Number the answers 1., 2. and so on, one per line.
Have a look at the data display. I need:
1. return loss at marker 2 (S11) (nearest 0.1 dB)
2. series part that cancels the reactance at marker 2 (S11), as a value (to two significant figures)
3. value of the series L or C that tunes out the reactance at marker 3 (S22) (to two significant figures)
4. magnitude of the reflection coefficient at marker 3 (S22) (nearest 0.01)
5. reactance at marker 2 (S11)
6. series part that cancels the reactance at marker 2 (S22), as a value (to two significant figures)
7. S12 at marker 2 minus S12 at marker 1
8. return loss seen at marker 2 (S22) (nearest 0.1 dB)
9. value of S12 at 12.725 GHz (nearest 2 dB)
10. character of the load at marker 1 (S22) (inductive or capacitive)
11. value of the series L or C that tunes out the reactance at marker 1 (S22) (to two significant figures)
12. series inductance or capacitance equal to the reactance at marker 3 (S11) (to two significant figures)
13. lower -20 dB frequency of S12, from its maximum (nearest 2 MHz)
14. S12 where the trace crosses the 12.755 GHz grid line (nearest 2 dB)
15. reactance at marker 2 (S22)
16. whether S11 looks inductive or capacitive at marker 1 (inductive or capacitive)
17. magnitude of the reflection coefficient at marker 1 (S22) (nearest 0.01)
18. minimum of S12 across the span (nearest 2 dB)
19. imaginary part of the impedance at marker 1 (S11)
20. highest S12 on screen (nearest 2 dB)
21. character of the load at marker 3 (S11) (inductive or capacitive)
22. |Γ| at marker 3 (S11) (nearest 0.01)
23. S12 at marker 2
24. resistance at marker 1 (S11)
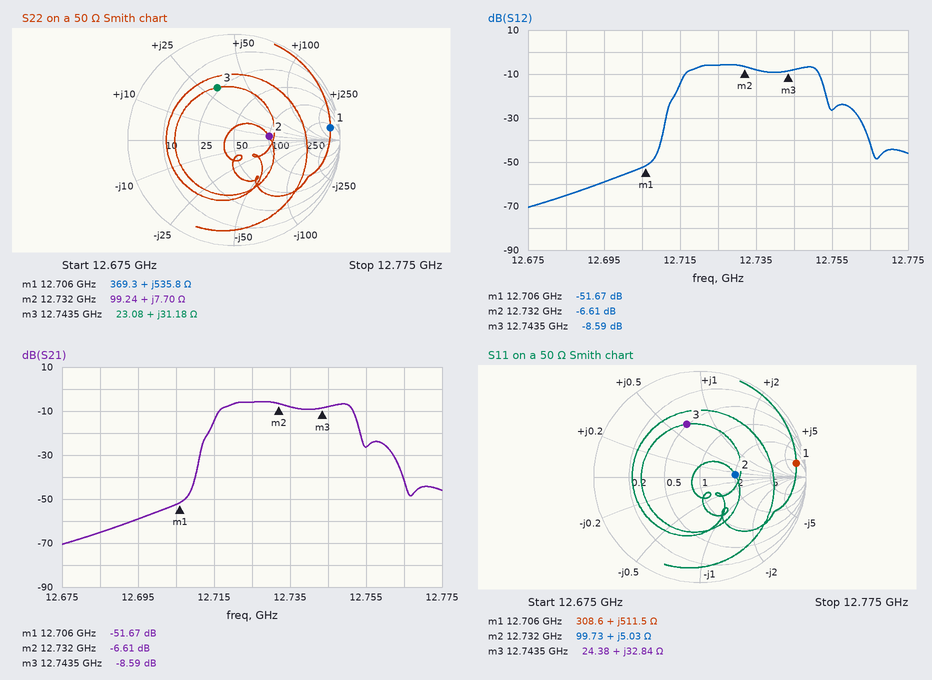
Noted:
1. 9.5 dB
2. 2.5 pF
3. 400 fF
4. 0.52
5. +5.03 Ω
6. 1.6 pF
7. 45.06 dB
8. 9.5 dB
9. -6 dB
10. inductive
11. 23 fF
12. 410 pH
13. 12.712 GHz
14. -26 dB
15. +7.70 Ω
16. inductive
17. 0.92
18. -70 dB
19. +511.5 Ω
20. -6 dB
21. inductive
22. 0.51
23. -6.61 dB
24. 308.6 Ω
